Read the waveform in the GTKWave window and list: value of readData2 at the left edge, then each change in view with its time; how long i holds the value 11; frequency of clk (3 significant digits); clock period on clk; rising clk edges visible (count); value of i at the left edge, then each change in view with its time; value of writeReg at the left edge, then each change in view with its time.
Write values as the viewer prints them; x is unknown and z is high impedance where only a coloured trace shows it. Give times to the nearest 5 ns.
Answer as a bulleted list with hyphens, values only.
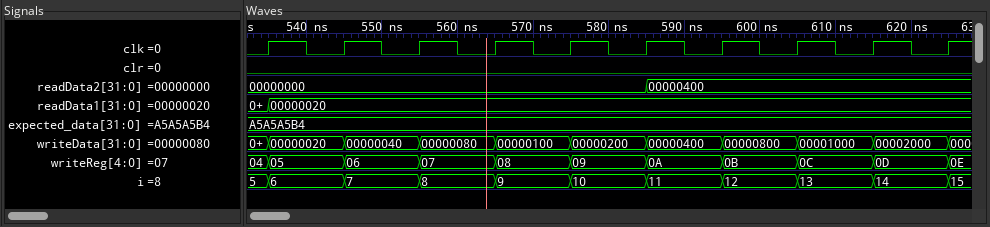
- 00000000, 00000400 at 585 ns
- 10 ns
- 100 MHz
- 10 ns
- 10
- 5, 6 at 535 ns, 7 at 545 ns, 8 at 555 ns, 9 at 565 ns, 10 at 575 ns, 11 at 585 ns, 12 at 595 ns, 13 at 605 ns, 14 at 615 ns, 15 at 625 ns
- 04, 05 at 535 ns, 06 at 545 ns, 07 at 555 ns, 08 at 565 ns, 09 at 575 ns, 0A at 585 ns, 0B at 595 ns, 0C at 605 ns, 0D at 615 ns, 0E at 625 ns
